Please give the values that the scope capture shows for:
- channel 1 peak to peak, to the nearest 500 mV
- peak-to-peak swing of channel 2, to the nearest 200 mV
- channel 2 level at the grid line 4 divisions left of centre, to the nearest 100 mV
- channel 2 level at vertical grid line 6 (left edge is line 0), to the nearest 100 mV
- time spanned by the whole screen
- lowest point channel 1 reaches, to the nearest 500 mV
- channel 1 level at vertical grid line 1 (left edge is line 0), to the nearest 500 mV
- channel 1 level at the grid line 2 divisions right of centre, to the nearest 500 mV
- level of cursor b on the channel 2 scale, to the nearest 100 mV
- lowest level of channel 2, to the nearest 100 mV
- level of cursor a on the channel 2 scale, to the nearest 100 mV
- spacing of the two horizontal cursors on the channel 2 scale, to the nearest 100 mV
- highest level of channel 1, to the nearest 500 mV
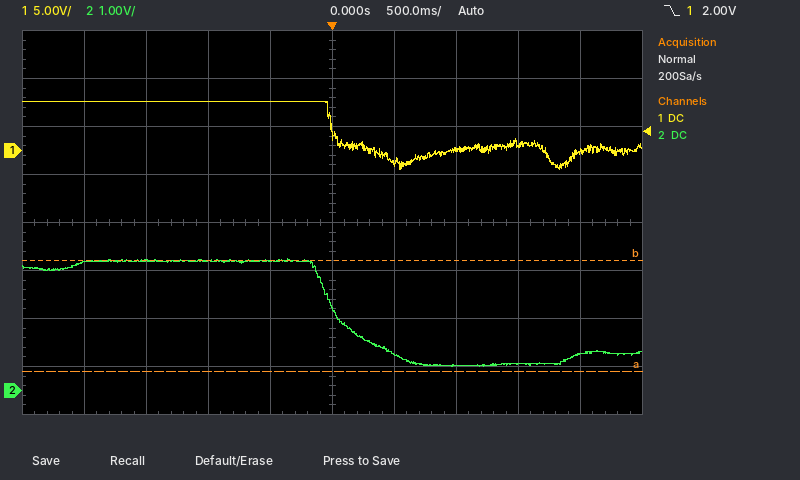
7.0 V
2.2 V
2.7 V
800 mV
5 s
-2.0 V
5.0 V
0.0 V
2.7 V
500 mV
400 mV
2.3 V
5.0 V
